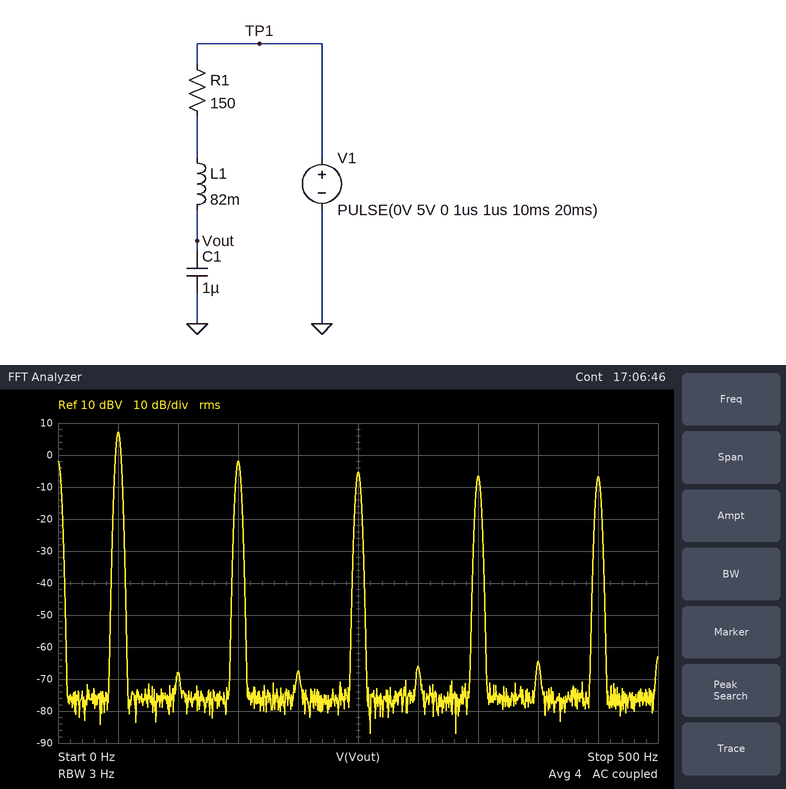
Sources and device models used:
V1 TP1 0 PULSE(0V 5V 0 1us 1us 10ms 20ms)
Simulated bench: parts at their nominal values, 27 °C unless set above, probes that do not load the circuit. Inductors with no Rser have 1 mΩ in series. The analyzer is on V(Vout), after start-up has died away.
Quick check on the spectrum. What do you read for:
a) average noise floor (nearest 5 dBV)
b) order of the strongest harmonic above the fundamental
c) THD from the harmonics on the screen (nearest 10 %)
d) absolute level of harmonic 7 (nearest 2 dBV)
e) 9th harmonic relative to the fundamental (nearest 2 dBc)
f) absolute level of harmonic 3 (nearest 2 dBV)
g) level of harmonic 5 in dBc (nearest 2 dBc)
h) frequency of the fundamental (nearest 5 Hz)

-75 dBV
3
50 %
-6 dBV
-14 dBc
-2 dBV
-12 dBc
50 Hz
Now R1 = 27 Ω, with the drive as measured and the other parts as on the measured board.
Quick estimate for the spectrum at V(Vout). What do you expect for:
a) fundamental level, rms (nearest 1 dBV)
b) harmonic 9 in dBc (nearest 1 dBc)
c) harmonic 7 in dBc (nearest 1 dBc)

7 dBV
-10 dBc
-13 dBc
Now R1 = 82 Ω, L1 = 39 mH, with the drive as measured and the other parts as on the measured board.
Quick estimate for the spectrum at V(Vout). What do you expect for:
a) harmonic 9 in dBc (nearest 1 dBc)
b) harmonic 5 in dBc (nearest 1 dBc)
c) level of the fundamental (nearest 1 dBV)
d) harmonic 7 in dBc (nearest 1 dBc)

-16 dBc
-13 dBc
7 dBV
-15 dBc
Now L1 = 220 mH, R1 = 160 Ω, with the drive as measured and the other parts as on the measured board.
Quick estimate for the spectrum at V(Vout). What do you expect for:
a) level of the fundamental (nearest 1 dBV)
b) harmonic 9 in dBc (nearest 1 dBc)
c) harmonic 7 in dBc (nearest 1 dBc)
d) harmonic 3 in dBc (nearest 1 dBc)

7 dBV
-18 dBc
-8 dBc
-8 dBc
